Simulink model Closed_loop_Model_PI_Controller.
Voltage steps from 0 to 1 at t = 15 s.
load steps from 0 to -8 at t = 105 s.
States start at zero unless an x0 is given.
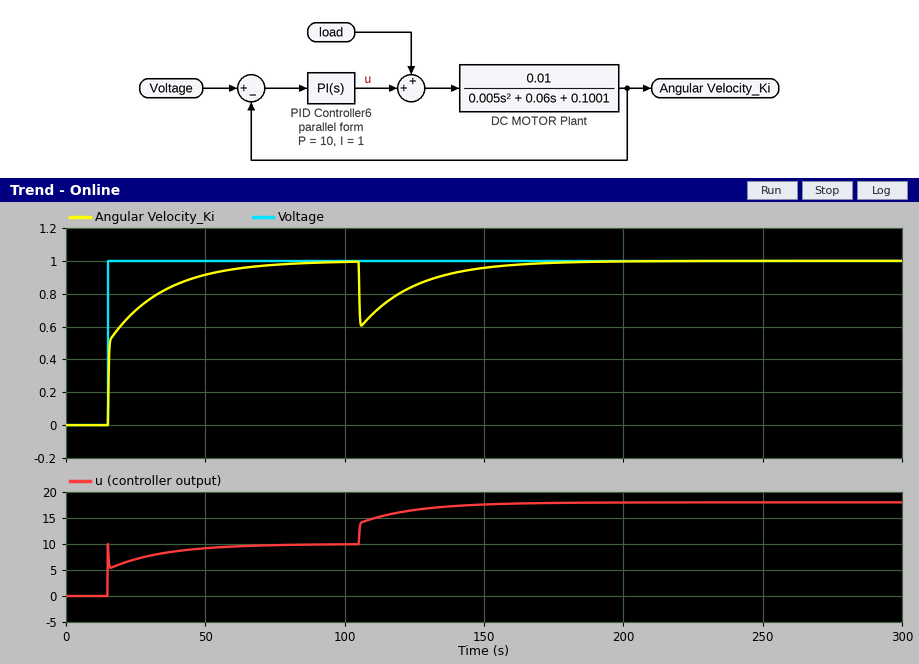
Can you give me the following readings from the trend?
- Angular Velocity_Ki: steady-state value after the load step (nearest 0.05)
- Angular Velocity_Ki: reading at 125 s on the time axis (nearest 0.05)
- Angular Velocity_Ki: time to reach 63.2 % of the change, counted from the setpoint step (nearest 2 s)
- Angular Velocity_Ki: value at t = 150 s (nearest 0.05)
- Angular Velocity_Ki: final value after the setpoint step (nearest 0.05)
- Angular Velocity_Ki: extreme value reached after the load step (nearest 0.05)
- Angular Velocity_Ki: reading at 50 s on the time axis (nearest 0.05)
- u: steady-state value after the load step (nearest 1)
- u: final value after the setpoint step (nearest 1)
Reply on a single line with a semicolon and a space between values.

1.00; 0.85; 6 s; 0.95; 1.00; 0.60; 0.90; 18; 10
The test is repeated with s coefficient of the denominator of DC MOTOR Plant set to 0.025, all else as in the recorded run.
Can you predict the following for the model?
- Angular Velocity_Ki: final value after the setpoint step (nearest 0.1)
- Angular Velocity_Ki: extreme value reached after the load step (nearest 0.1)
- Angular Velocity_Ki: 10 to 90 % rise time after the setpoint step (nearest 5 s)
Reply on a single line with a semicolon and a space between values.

1.0; 0.5; 30 s
